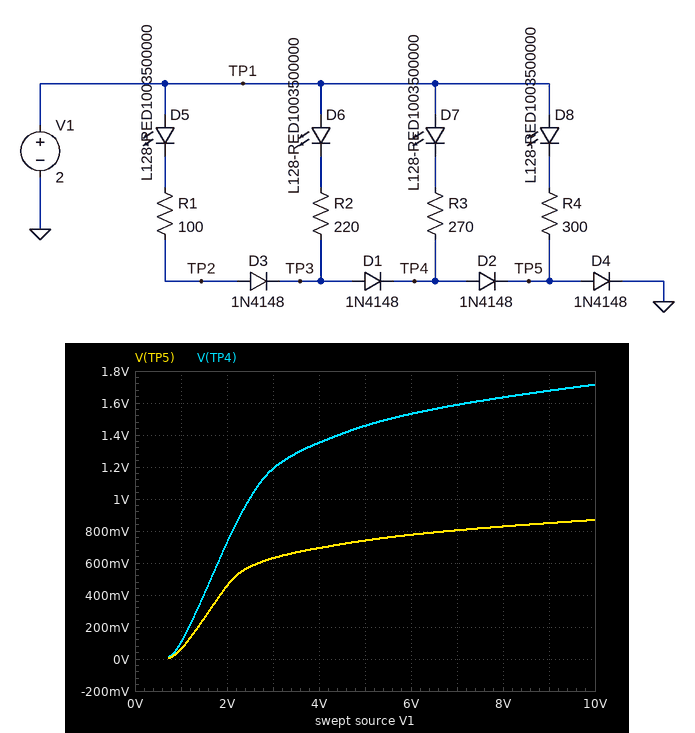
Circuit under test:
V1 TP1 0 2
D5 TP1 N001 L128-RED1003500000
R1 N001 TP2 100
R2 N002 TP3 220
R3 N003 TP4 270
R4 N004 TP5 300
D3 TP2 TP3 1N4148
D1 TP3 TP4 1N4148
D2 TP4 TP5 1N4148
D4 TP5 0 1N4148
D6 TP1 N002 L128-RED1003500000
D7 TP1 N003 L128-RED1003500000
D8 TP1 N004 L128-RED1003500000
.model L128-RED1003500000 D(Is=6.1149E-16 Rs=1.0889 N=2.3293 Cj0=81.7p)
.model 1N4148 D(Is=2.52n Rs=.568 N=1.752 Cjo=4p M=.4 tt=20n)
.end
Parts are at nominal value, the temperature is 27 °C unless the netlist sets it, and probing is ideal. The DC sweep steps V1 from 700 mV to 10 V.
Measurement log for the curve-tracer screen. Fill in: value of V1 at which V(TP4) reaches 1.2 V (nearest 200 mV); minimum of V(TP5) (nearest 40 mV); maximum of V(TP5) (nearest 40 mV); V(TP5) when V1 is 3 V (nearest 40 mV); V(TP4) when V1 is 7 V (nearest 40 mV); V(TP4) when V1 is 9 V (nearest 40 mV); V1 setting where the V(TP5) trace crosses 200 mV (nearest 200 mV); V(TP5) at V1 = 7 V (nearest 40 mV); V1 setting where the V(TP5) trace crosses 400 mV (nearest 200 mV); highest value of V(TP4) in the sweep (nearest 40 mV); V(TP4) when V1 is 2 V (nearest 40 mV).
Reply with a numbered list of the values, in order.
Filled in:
1. 3.0 V
2. 0 V
3. 880 mV
4. 640 mV
5. 1.60 V
6. 1.68 V
7. 1.4 V
8. 800 mV
9. 1.8 V
10. 1.72 V
11. 720 mV
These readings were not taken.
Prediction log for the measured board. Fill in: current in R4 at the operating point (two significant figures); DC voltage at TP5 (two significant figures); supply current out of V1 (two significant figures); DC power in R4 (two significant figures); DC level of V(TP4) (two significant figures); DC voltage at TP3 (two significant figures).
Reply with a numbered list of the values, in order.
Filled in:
1. 60 µA
2. 460 mV
3. 61 µA
4. 1.1 µW
5. 730 mV
6. 890 mV
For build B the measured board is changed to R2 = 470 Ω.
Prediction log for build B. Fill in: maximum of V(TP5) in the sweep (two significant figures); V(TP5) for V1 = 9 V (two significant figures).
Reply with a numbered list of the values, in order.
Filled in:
1. 860 mV
2. 840 mV
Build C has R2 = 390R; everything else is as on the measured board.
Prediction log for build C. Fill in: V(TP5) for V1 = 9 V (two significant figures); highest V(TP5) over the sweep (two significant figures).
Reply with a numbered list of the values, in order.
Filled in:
1. 840 mV
2. 860 mV
